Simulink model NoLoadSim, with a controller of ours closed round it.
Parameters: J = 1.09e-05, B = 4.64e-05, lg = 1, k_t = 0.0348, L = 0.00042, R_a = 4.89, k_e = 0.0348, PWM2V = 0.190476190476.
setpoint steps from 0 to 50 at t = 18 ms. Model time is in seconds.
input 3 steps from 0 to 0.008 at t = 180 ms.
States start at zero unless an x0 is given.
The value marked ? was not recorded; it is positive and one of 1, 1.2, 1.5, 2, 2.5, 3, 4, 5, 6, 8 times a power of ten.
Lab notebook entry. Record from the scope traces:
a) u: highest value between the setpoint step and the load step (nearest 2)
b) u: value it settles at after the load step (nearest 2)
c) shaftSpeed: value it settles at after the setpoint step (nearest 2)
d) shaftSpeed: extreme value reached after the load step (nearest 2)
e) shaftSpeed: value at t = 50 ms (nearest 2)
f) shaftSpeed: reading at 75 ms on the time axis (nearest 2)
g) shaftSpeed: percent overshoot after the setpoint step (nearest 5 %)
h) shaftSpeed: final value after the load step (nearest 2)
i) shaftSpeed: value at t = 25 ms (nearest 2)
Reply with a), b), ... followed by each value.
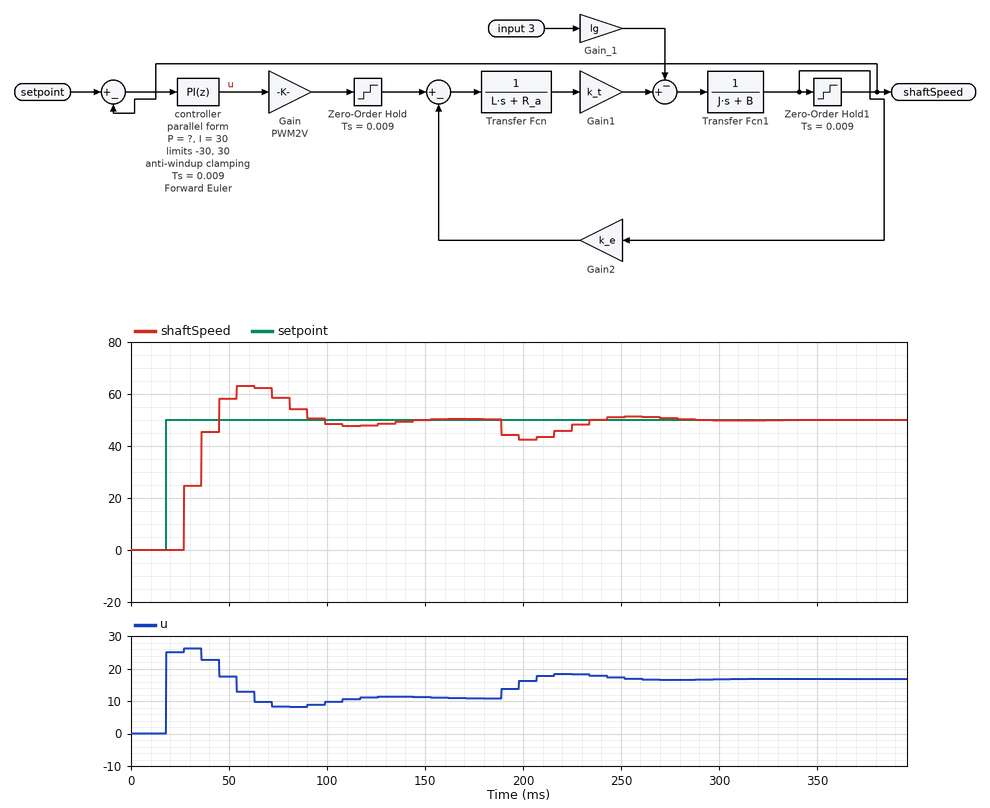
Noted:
a) 26
b) 16
c) 50
d) 42
e) 58
f) 58
g) 25 %
h) 50
i) 0
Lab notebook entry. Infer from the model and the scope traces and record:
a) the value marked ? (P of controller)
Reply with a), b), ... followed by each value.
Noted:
a) 0.5
